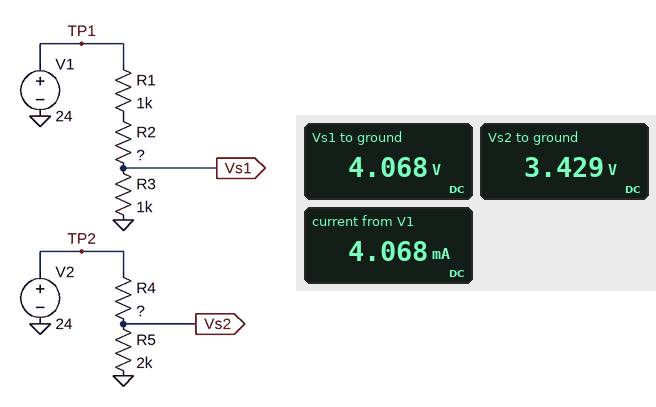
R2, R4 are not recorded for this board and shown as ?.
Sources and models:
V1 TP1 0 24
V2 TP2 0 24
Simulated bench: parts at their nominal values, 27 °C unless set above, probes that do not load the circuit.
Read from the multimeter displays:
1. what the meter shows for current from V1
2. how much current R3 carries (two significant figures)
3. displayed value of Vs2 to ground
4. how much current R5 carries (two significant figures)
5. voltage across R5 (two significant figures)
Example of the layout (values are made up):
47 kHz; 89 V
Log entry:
4.068 mA; 4.1 mA; 3.429 V; 1.7 mA; 3.4 V
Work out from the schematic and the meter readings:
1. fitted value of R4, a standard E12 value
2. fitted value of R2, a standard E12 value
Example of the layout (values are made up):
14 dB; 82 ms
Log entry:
12 kΩ; 3.9 kΩ
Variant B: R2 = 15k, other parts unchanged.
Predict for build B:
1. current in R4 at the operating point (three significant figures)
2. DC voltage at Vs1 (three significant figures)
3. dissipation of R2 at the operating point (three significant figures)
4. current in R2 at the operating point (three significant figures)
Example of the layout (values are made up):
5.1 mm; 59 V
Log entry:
1.71 mA; 1.41 V; 29.9 mW; 1.41 mA
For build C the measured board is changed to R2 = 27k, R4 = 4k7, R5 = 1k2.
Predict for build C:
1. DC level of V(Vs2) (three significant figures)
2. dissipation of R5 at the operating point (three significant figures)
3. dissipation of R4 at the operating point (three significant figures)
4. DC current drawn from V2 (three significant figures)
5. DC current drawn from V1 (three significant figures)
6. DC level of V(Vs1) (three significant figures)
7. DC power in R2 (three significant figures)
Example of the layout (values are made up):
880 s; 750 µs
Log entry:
4.88 V; 19.9 mW; 77.8 mW; 4.07 mA; 828 µA; 828 mV; 18.5 mW
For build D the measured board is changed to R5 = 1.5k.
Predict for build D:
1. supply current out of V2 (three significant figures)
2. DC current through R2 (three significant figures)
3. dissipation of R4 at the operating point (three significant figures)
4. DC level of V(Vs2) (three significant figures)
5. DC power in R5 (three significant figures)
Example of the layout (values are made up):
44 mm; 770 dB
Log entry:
1.78 mA; 4.07 mA; 37.9 mW; 2.67 V; 4.74 mW
